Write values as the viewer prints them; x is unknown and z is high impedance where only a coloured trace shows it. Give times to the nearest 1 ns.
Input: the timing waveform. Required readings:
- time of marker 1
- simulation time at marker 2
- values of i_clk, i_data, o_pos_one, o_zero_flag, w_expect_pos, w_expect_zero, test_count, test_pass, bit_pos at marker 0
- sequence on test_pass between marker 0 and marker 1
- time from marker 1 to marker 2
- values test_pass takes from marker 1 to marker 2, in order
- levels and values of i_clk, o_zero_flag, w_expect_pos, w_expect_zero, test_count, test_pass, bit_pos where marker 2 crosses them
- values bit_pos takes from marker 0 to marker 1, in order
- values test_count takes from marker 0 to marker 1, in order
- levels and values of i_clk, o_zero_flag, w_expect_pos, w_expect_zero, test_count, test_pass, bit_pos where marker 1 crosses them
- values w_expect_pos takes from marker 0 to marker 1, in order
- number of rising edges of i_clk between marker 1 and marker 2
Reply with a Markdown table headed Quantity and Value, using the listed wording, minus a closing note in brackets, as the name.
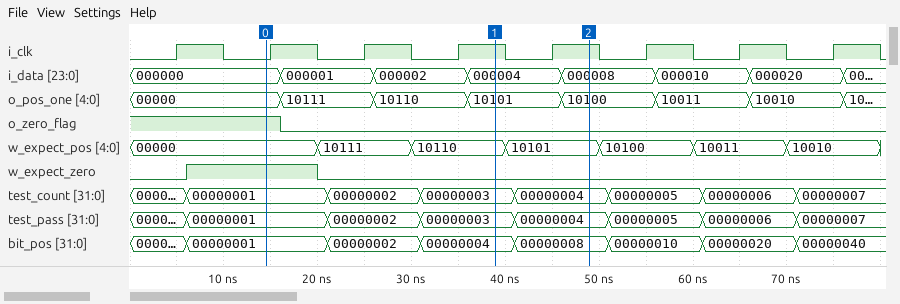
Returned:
| Quantity | Value |
|---|---|
| time of marker 1 | 39 ns |
| simulation time at marker 2 | 49 ns |
| values of i_clk, i_data, o_pos_one, o_zero_flag, w_expect_pos, w_expect_zero, test_count, test_pass, bit_pos at marker 0 | i_clk=0, i_data=000000, o_pos_one=00000, o_zero_flag=1, w_expect_pos=00000, w_expect_zero=1, test_count=00000001, test_pass=00000001, bit_pos=00000001 |
| sequence on test_pass between marker 0 and marker 1 | 00000001, 00000002, 00000003 |
| time from marker 1 to marker 2 | 10 ns |
| values test_pass takes from marker 1 to marker 2, in order | 00000003, 00000004 |
| levels and values of i_clk, o_zero_flag, w_expect_pos, w_expect_zero, test_count, test_pass, bit_pos where marker 2 crosses them | i_clk=1, o_zero_flag=0, w_expect_pos=10101, w_expect_zero=0, test_count=00000004, test_pass=00000004, bit_pos=00000008 |
| values bit_pos takes from marker 0 to marker 1, in order | 00000001, 00000002, 00000004 |
| values test_count takes from marker 0 to marker 1, in order | 00000001, 00000002, 00000003 |
| levels and values of i_clk, o_zero_flag, w_expect_pos, w_expect_zero, test_count, test_pass, bit_pos where marker 1 crosses them | i_clk=1, o_zero_flag=0, w_expect_pos=10110, w_expect_zero=0, test_count=00000003, test_pass=00000003, bit_pos=00000004 |
| values w_expect_pos takes from marker 0 to marker 1, in order | 00000, 10111, 10110 |
| number of rising edges of i_clk between marker 1 and marker 2 | 1 |
